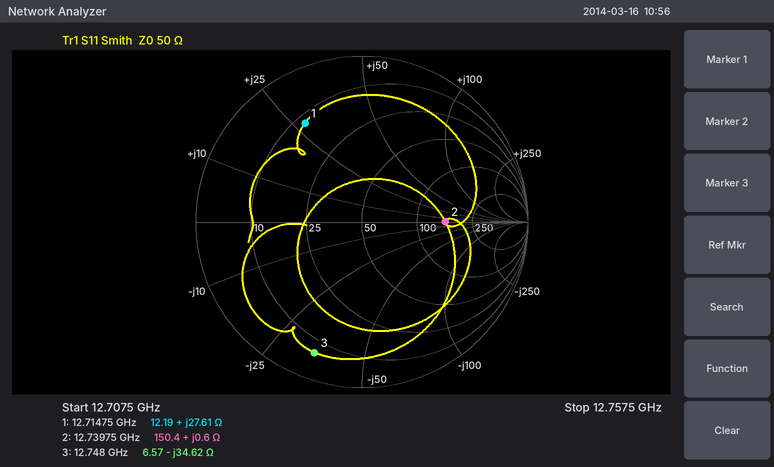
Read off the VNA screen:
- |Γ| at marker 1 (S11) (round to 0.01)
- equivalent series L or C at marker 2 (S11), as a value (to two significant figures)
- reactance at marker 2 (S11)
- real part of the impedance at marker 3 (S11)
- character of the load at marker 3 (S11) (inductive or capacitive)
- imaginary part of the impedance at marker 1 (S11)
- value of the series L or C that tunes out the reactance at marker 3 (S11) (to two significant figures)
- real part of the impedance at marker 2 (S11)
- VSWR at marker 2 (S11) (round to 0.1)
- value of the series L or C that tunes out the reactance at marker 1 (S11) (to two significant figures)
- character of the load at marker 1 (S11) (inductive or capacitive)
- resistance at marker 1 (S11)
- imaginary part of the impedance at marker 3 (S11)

0.69
7.5 pH
+0.6 Ω
6.57 Ω
capacitive
+27.61 Ω
430 pH
150.4 Ω
3.0
450 fF
inductive
12.19 Ω
-34.62 Ω
